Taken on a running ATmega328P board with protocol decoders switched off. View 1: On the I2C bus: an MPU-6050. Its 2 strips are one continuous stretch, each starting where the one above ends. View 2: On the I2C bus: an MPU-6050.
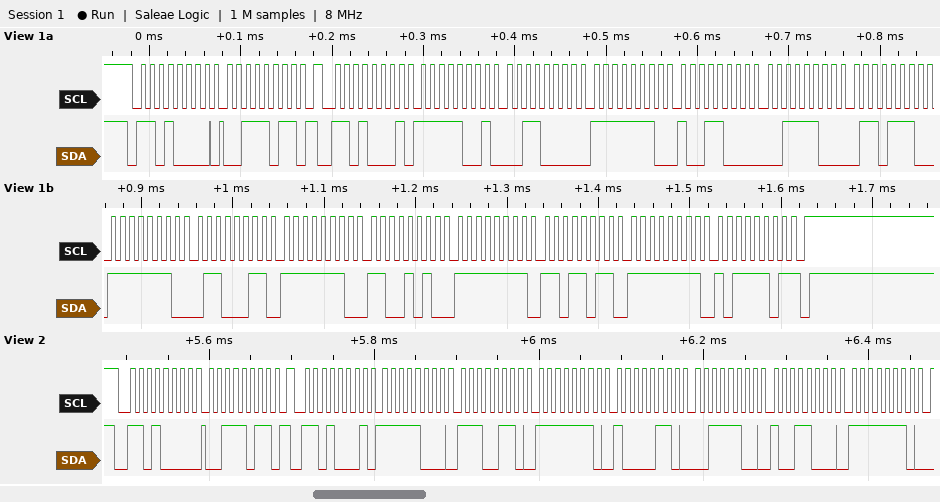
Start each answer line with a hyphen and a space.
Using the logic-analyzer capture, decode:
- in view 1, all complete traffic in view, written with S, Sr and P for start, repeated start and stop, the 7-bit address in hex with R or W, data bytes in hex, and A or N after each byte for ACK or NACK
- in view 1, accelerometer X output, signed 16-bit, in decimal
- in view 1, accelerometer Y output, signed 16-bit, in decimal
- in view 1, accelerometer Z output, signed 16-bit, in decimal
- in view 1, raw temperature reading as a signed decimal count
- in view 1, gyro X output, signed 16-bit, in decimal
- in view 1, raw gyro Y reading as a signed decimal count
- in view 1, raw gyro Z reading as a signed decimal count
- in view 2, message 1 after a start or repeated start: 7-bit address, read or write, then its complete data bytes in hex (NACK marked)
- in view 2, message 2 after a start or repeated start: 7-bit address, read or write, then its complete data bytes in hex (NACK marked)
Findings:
- S 68W A 3B A Sr 68R A F9 A 30 A FE A 98 A 3C A 6E A FE A 63 A FE A CA A FF A DB A FF A BD N P
- -1744
- -360
- 15470
- -413
- -310
- -37
- -67
- 0x68 write: 3B
- 0x68 read: F8 E6 FE 86 3C 98 FE
